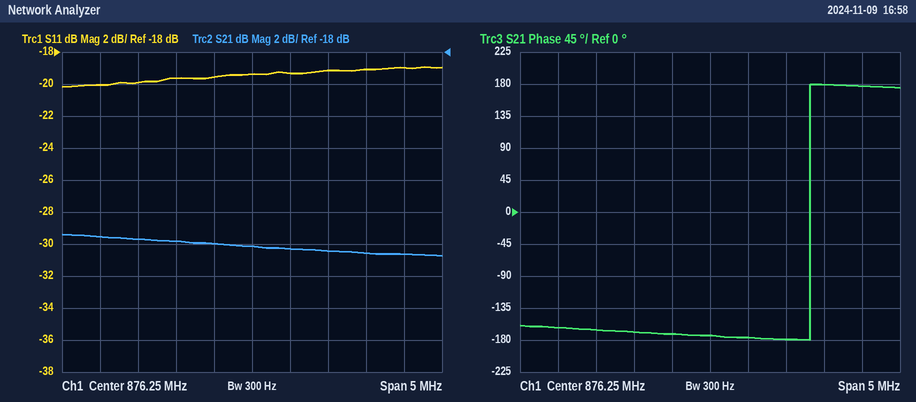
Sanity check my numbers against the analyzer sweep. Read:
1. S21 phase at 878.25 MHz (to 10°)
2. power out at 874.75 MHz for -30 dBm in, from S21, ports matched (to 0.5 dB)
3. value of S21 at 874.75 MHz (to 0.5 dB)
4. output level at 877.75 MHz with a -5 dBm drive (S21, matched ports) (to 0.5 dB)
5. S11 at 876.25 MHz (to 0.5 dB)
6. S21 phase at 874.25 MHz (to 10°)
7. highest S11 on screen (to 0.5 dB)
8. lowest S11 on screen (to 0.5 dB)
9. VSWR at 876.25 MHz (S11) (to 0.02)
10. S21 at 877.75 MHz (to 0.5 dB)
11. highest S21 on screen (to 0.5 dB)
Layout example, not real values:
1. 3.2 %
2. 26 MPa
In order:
1. 180°
2. -59.5 dBm
3. -29.5 dB
4. -35.5 dBm
5. -19.5 dB
6. -160°
7. -19.0 dB
8. -20.0 dB
9. 1.24
10. -30.5 dB
11. -29.5 dB
